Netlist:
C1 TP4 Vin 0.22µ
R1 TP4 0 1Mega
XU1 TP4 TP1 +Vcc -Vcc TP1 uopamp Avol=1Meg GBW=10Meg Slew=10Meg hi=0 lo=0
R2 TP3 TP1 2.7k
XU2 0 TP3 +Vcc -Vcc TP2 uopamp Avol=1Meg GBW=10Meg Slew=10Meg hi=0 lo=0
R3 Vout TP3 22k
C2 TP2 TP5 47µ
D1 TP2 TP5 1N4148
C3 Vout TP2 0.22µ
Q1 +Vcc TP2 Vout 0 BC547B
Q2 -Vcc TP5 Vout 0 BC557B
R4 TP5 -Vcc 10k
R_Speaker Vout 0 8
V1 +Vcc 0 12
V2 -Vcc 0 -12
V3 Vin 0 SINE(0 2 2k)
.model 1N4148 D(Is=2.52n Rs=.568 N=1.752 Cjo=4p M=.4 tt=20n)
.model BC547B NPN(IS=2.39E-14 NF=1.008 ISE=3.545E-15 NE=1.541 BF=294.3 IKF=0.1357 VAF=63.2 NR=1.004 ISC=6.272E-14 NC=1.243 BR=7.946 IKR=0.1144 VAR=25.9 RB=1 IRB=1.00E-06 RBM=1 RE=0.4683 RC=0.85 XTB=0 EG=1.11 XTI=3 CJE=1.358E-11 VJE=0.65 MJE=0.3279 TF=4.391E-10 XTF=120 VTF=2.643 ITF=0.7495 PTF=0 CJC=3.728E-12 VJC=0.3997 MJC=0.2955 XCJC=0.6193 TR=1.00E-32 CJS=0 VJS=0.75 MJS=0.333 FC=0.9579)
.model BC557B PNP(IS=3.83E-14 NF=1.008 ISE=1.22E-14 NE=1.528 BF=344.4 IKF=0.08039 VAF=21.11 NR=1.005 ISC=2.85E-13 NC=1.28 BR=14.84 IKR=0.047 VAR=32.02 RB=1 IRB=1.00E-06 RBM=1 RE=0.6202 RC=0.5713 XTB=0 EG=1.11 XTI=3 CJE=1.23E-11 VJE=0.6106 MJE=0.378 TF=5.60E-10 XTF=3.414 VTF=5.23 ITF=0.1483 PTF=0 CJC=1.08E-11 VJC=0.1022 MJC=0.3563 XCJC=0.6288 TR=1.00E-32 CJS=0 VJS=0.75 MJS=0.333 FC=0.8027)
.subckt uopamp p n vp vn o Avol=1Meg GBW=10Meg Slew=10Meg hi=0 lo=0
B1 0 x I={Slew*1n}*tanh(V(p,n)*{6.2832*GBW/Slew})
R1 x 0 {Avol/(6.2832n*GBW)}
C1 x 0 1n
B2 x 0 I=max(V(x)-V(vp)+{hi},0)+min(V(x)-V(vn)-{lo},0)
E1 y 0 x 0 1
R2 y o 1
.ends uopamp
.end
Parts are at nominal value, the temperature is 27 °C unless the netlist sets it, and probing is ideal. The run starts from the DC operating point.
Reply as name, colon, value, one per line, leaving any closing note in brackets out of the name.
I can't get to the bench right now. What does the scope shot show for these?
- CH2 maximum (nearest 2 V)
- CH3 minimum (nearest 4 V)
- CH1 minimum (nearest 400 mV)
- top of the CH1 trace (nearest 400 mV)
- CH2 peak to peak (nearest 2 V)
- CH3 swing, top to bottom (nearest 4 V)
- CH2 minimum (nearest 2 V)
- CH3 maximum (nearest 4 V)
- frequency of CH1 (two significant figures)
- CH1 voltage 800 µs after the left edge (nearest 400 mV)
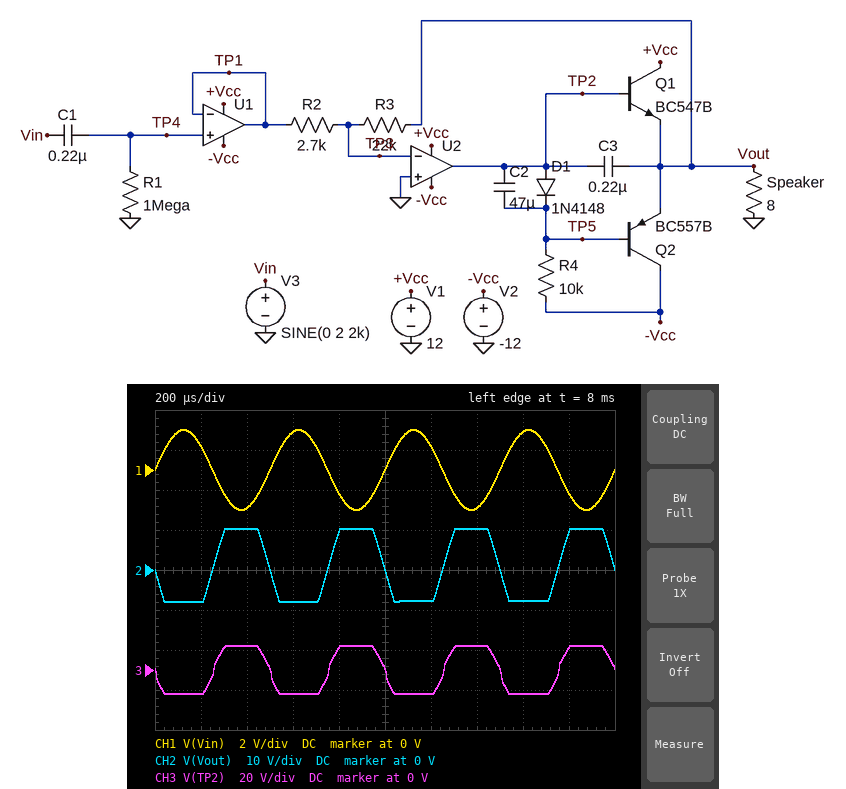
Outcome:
CH2 maximum: 10 V
CH3 minimum: -12 V
CH1 minimum: -2.0 V
top of the CH1 trace: 2.0 V
CH2 peak to peak: 18 V
CH3 swing, top to bottom: 24 V
CH2 minimum: -8 V
CH3 maximum: 12 V
frequency of CH1: 2.0 kHz
CH1 voltage 800 µs after the left edge: -1.2 V
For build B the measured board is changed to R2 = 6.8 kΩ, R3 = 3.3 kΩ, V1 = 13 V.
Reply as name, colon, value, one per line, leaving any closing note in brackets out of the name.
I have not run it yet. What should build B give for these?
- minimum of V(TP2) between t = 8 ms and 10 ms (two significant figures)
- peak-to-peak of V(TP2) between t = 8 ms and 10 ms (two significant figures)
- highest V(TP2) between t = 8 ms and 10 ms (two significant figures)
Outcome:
minimum of V(TP2) between t = 8 ms and 10 ms: -1.2 V
peak-to-peak of V(TP2) between t = 8 ms and 10 ms: 3.0 V
highest V(TP2) between t = 8 ms and 10 ms: 1.8 V
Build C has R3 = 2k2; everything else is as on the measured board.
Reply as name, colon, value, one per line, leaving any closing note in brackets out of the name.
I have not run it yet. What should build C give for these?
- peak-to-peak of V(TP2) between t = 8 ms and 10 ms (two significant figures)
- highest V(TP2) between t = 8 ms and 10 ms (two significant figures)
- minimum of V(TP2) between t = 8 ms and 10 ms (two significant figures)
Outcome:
peak-to-peak of V(TP2) between t = 8 ms and 10 ms: 4.5 V
highest V(TP2) between t = 8 ms and 10 ms: 2.5 V
minimum of V(TP2) between t = 8 ms and 10 ms: -2.0 V
